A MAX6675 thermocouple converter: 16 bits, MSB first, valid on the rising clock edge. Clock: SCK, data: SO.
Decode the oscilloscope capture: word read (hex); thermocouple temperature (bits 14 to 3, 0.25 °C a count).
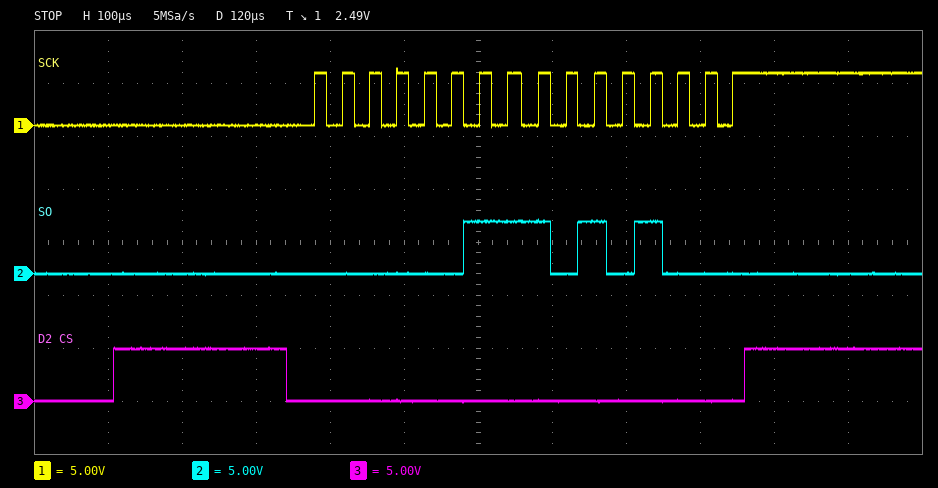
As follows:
0x03A8
29.25 °C
